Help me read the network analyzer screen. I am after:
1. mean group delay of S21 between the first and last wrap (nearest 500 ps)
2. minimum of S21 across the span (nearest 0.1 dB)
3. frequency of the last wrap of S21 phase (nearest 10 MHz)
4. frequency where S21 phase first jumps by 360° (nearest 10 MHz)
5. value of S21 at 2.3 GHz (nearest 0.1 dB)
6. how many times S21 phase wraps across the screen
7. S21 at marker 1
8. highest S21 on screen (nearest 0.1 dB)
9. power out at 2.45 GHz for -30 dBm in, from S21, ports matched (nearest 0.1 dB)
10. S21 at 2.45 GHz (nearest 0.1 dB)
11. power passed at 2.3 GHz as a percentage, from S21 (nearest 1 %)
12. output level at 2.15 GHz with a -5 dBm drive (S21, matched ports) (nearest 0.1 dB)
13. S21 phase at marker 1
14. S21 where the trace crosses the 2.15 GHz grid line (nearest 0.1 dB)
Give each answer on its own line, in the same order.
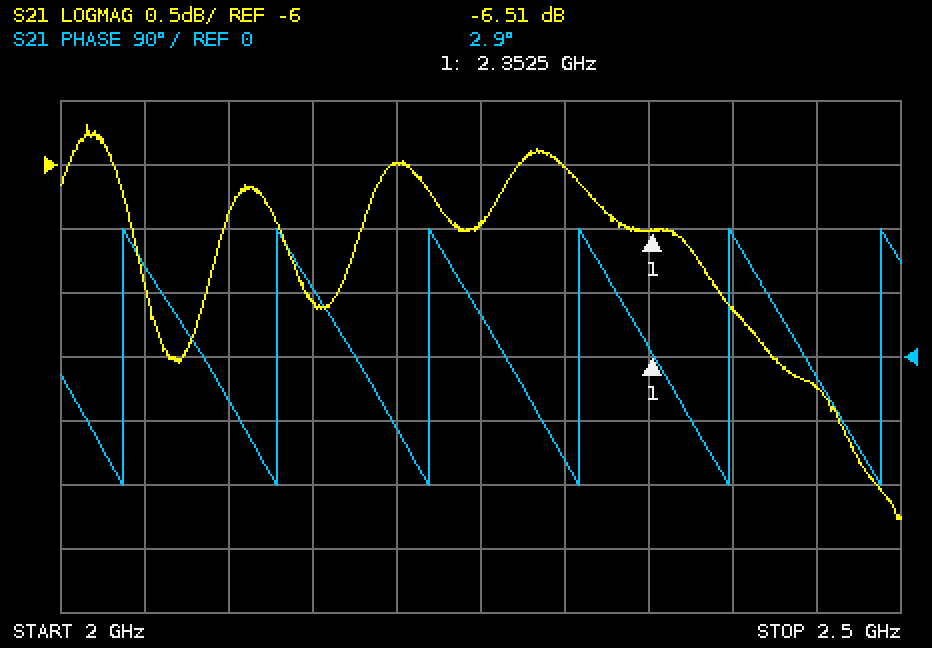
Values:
11.0 ns
-8.8 dB
2.49 GHz
2.04 GHz
-6.0 dB
6
-6.51 dB
-5.7 dB
-37.7 dBm
-7.7 dB
25 %
-12.1 dBm
2.9°
-7.1 dB
